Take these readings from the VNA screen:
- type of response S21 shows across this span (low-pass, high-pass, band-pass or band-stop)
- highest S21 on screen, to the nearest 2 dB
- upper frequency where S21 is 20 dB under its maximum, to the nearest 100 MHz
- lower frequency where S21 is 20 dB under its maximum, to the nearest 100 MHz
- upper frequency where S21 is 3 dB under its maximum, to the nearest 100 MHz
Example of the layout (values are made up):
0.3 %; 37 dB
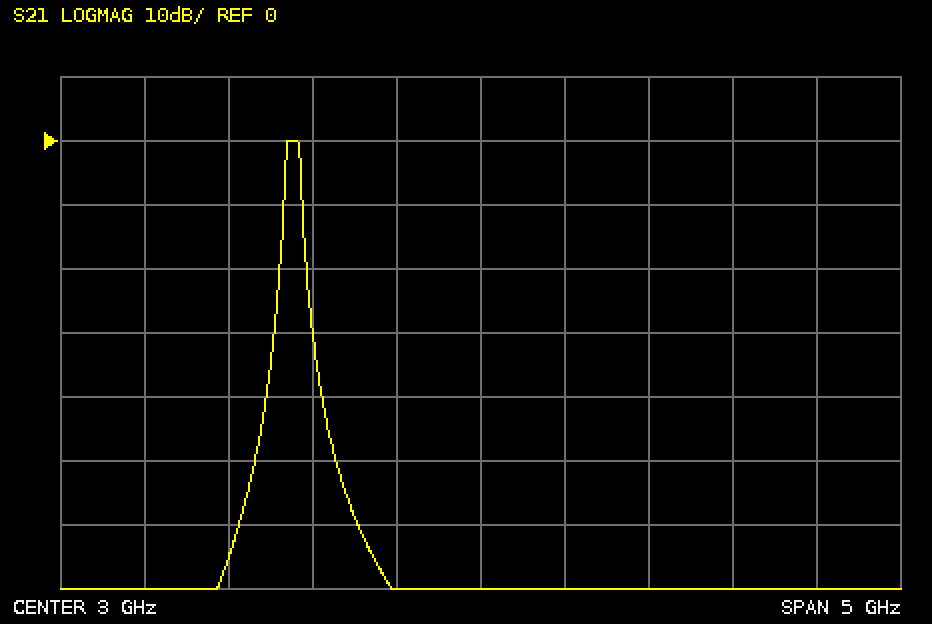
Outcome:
band-pass; 0 dB; 2.0 GHz; 1.8 GHz; 1.9 GHz
